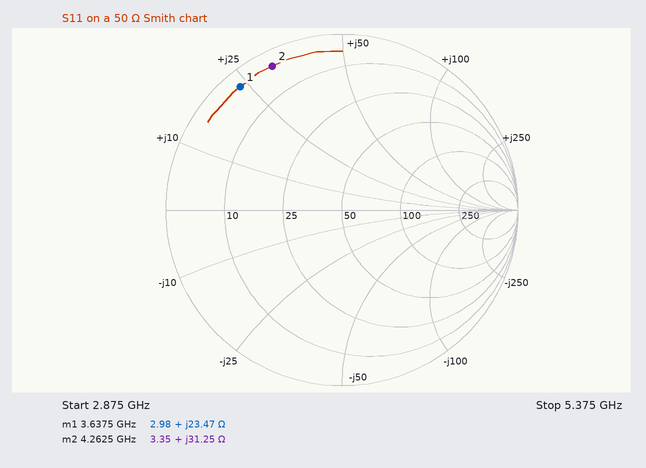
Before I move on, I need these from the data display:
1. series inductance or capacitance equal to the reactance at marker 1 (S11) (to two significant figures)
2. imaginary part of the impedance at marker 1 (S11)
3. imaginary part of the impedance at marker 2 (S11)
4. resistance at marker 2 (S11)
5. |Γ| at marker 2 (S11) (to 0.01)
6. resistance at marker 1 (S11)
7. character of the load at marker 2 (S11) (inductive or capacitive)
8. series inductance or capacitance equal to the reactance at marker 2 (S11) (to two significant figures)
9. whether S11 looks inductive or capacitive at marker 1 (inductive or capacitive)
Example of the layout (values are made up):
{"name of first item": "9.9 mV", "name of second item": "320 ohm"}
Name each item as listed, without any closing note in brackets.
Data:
{"series inductance or capacitance equal to the reactance at marker 1 (S11)": "1.0 nH", "imaginary part of the impedance at marker 1": "+23.47 Ω", "imaginary part of the impedance at marker 2": "+31.25 Ω", "resistance at marker 2": "3.35 Ω", "|Γ| at marker 2 (S11)": "0.91", "resistance at marker 1": "2.98 Ω", "character of the load at marker 2 (S11)": "inductive", "series inductance or capacitance equal to the reactance at marker 2 (S11)": "1.2 nH", "whether S11 looks inductive or capacitive at marker 1": "inductive"}
